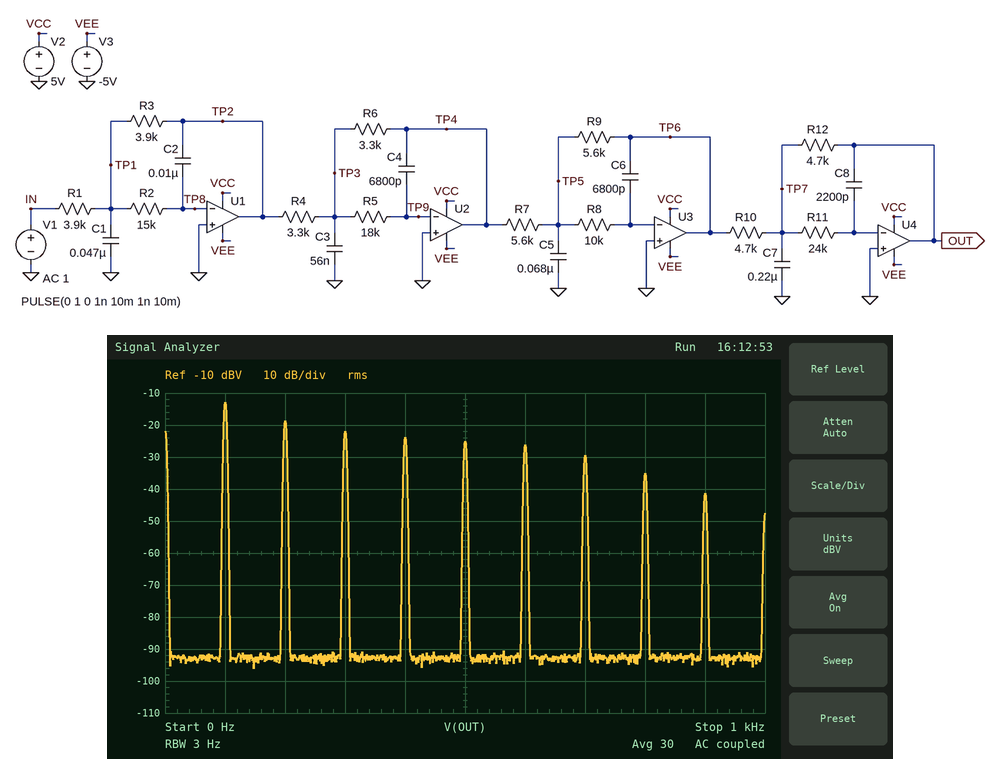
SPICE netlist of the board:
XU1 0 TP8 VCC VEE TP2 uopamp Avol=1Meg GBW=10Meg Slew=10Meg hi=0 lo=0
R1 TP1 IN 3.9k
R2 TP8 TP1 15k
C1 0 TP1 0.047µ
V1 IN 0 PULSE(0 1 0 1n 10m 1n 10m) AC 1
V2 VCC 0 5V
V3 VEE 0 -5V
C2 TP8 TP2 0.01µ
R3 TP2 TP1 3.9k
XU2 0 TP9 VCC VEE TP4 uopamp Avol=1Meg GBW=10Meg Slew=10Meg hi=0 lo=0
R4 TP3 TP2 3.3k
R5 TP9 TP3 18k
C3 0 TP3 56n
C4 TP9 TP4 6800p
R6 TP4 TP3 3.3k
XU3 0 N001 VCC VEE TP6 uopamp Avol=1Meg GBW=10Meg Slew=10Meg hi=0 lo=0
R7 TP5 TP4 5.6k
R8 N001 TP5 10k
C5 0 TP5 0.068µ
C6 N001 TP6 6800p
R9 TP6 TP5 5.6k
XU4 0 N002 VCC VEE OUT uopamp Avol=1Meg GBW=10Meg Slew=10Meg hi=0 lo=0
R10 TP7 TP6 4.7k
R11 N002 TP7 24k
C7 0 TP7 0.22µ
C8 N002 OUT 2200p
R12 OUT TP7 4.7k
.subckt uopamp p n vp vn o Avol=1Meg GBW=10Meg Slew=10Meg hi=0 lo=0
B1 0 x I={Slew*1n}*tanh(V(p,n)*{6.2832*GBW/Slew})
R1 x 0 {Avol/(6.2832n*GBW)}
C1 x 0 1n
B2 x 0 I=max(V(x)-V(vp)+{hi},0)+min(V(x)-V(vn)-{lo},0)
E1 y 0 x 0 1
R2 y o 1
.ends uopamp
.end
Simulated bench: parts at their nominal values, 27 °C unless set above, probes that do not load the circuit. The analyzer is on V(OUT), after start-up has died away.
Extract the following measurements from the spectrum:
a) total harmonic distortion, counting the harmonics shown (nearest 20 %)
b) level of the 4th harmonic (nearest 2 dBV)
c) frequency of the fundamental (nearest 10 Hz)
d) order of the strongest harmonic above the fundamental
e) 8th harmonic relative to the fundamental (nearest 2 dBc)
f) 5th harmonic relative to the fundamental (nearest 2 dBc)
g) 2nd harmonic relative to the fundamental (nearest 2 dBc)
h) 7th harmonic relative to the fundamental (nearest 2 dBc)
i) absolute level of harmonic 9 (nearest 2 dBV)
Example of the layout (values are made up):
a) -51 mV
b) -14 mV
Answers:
a) 80 %
b) -24 dBV
c) 100 Hz
d) 2
e) -22 dBc
f) -12 dBc
g) -6 dBc
h) -16 dBc
i) -42 dBV
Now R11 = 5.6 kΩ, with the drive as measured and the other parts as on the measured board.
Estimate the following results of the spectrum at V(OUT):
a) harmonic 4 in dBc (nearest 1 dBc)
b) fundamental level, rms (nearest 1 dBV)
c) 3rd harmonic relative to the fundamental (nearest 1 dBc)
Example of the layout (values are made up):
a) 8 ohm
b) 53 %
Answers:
a) -13 dBc
b) -13 dBV
c) -10 dBc
